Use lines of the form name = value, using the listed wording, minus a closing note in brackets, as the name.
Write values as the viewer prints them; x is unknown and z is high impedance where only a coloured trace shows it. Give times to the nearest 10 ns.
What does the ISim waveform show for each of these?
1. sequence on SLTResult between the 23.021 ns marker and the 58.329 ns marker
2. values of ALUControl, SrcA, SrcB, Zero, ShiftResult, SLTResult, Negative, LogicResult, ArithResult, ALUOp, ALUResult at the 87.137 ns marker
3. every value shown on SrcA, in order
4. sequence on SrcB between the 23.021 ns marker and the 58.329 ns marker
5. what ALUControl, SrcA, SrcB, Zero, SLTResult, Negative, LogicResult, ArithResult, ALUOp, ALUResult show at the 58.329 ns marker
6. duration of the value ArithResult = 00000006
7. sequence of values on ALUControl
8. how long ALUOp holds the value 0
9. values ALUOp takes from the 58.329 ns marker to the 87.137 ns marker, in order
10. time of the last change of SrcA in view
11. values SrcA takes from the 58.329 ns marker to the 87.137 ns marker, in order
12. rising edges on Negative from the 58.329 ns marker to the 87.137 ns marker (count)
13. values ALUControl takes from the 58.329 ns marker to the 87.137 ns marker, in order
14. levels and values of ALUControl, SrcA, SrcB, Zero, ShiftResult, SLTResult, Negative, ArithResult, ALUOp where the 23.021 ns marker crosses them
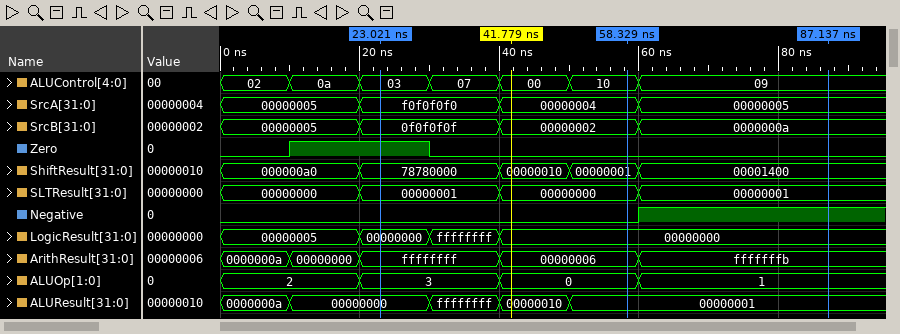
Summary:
sequence on SLTResult between the 23.021 ns marker and the 58.329 ns marker = 00000001, 00000000
values of ALUControl, SrcA, SrcB, Zero, ShiftResult, SLTResult, Negative, LogicResult, ArithResult, ALUOp, ALUResult at the 87.137 ns marker = ALUControl=09, SrcA=00000005, SrcB=0000000a, Zero=0, ShiftResult=00001400, SLTResult=00000001, Negative=1, LogicResult=00000000, ArithResult=fffffffb, ALUOp=1, ALUResult=00000001
every value shown on SrcA, in order = 00000005, f0f0f0f0, 00000004, 00000005
sequence on SrcB between the 23.021 ns marker and the 58.329 ns marker = 0f0f0f0f, 00000002
what ALUControl, SrcA, SrcB, Zero, SLTResult, Negative, LogicResult, ArithResult, ALUOp, ALUResult show at the 58.329 ns marker = ALUControl=10, SrcA=00000004, SrcB=00000002, Zero=0, SLTResult=00000000, Negative=0, LogicResult=00000000, ArithResult=00000006, ALUOp=0, ALUResult=00000001
duration of the value ArithResult = 00000006 = 20 ns
sequence of values on ALUControl = 02, 0a, 03, 07, 00, 10, 09
how long ALUOp holds the value 0 = 20 ns
values ALUOp takes from the 58.329 ns marker to the 87.137 ns marker, in order = 0, 1
time of the last change of SrcA in view = 60 ns
values SrcA takes from the 58.329 ns marker to the 87.137 ns marker, in order = 00000004, 00000005
rising edges on Negative from the 58.329 ns marker to the 87.137 ns marker = 1
values ALUControl takes from the 58.329 ns marker to the 87.137 ns marker, in order = 10, 09
levels and values of ALUControl, SrcA, SrcB, Zero, ShiftResult, SLTResult, Negative, ArithResult, ALUOp where the 23.021 ns marker crosses them = ALUControl=03, SrcA=f0f0f0f0, SrcB=0f0f0f0f, Zero=1, ShiftResult=78780000, SLTResult=00000001, Negative=0, ArithResult=ffffffff, ALUOp=3
